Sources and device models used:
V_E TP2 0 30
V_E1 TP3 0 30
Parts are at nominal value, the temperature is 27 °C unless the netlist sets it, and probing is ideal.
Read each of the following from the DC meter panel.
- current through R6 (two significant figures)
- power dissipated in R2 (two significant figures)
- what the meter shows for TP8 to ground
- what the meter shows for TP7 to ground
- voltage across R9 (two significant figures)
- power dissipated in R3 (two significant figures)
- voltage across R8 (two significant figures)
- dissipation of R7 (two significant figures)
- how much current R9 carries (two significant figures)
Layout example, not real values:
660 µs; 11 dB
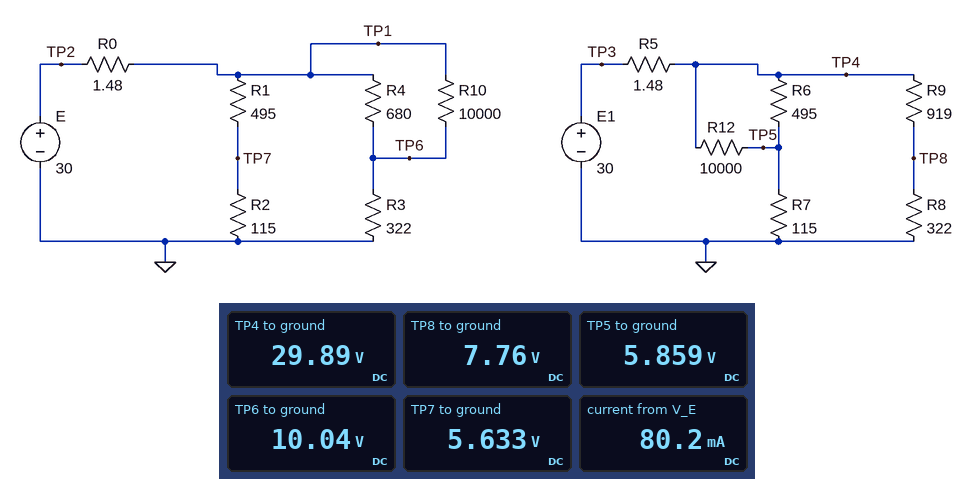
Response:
49 mA; 280 mW; 7.76 V; 5.633 V; 22 V; 310 mW; 7.8 V; 300 mW; 24 mA
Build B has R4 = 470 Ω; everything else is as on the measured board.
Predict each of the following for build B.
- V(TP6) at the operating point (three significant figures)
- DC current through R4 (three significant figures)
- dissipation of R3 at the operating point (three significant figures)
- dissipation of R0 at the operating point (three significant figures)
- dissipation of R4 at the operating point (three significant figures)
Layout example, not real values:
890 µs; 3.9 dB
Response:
12.5 V; 37.0 mA; 483 mW; 11.4 mW; 644 mW
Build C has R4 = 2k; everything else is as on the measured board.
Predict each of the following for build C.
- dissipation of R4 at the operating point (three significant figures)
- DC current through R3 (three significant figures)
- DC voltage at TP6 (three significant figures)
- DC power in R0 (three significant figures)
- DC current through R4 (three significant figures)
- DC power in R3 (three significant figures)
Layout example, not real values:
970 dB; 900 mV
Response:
314 mW; 15.0 mA; 4.84 V; 6.07 mW; 12.5 mA; 72.8 mW
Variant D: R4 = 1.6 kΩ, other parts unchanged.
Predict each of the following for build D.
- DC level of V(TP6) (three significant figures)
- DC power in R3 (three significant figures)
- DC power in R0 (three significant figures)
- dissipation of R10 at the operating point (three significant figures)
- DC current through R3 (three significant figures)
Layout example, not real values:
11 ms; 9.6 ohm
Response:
5.66 V; 99.5 mW; 6.56 mW; 58.8 mW; 17.6 mA
